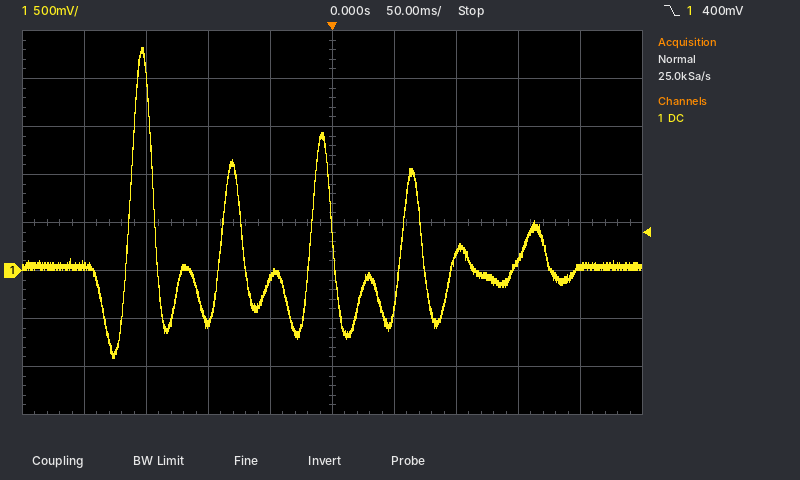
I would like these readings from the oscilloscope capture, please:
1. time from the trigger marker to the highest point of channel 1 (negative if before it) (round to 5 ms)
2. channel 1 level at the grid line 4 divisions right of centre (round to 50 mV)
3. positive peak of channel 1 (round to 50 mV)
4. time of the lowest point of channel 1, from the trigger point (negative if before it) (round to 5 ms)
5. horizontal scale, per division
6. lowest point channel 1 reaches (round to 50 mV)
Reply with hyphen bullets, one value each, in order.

- -155 ms
- 50 mV
- 2.30 V
- -175 ms
- 50 ms
- -900 mV
